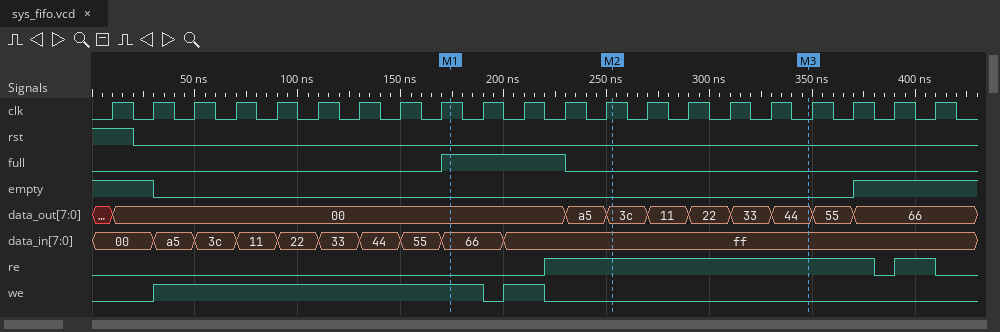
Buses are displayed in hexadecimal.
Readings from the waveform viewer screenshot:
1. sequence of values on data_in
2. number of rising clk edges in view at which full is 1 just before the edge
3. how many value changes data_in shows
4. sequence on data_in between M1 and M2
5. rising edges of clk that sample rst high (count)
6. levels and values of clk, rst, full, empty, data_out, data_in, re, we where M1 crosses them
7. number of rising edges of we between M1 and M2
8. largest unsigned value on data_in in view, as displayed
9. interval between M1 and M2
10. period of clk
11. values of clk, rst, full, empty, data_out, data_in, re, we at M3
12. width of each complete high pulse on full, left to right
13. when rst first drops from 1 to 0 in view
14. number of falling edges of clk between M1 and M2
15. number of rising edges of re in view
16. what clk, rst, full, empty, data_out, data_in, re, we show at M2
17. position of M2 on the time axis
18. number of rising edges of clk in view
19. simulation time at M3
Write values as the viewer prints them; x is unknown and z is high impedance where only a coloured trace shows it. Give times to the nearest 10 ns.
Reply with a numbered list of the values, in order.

1. 00, a5, 3c, 11, 22, 33, 44, 55, 66, ff
2. 3
3. 9
4. 66, ff
5. 1
6. clk=1, rst=0, full=1, empty=0, data_out=00, data_in=66, re=0, we=1
7. 1
8. ff
9. 80 ns
10. 20 ns
11. clk=0, rst=0, full=0, empty=0, data_out=44, data_in=ff, re=1, we=0
12. 60 ns
13. 20 ns
14. 4
15. 2
16. clk=1, rst=0, full=0, empty=0, data_out=3c, data_in=ff, re=1, we=0
17. 250 ns
18. 21
19. 350 ns
